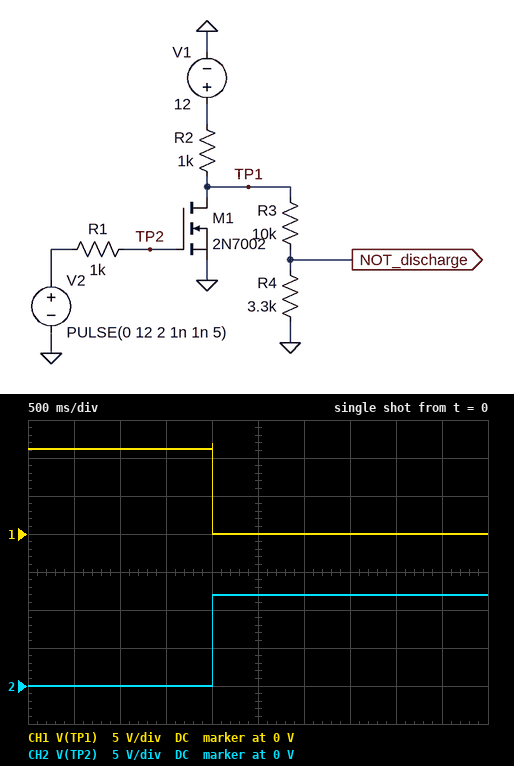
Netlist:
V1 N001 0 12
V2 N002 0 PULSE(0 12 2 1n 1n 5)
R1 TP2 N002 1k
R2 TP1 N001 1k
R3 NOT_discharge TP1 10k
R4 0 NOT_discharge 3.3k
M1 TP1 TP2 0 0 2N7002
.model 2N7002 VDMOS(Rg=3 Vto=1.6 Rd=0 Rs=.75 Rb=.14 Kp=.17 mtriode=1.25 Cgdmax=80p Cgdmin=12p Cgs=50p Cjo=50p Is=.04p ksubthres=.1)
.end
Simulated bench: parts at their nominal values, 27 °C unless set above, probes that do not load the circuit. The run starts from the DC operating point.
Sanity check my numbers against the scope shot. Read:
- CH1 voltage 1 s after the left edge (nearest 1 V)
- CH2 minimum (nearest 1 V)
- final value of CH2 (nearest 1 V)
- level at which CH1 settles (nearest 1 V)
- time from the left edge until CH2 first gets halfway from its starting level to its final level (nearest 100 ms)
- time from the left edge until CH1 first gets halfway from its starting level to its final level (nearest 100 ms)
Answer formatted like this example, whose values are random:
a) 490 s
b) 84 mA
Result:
a) 11 V
b) 0 V
c) 12 V
d) 0 V
e) 2.0 s
f) 2.0 s
